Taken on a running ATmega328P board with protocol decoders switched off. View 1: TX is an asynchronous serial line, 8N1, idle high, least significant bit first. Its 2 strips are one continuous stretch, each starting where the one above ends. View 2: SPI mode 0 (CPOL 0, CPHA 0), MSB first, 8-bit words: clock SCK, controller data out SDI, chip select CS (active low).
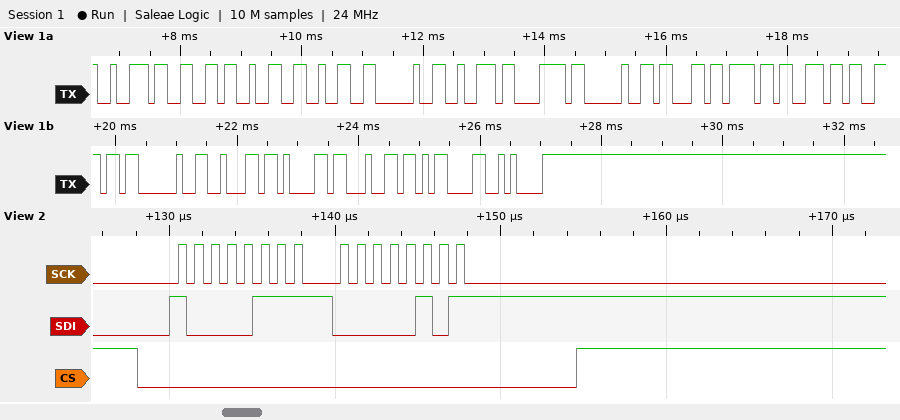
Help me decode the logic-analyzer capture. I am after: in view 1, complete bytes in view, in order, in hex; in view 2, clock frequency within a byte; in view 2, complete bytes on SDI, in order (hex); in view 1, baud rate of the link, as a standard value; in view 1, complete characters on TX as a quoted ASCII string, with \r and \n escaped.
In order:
72 66 32 32 20 72 78 20 63 6F 6E 6E 20 62 61 64 0D 0A
1 MHz
87 05
9600 baud
"rf22 rx conn bad\r\n"
